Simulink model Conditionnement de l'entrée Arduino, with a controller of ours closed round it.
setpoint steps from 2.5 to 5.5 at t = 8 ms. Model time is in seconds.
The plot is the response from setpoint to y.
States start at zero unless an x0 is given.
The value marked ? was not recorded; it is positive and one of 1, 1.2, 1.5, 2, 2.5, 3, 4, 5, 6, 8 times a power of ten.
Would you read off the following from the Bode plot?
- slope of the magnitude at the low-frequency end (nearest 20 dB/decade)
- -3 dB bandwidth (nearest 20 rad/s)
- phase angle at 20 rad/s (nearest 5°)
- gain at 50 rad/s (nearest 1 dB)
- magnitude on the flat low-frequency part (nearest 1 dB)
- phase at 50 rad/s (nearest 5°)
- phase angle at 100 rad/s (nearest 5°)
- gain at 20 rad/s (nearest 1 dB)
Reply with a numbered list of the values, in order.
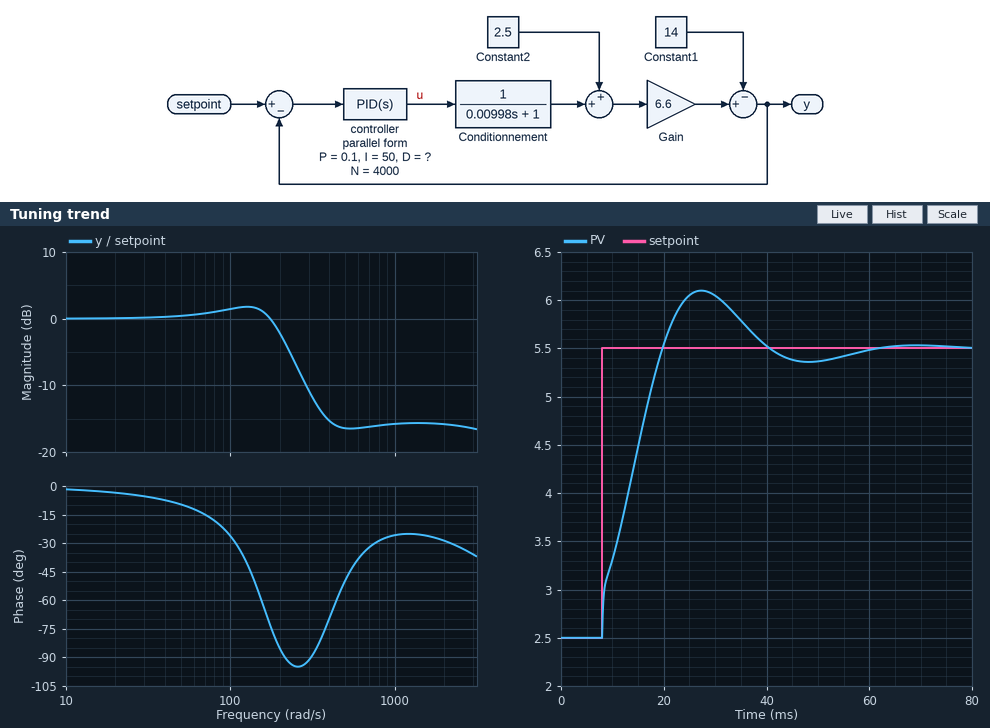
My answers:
1. 0 dB/decade
2. 200 rad/s
3. -5°
4. 0 dB
5. 0 dB
6. -10°
7. -25°
8. 0 dB
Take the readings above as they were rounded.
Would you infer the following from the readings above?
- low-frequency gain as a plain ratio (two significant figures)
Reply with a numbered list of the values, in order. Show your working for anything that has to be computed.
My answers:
1. 10^(0 / 20) = 1.0
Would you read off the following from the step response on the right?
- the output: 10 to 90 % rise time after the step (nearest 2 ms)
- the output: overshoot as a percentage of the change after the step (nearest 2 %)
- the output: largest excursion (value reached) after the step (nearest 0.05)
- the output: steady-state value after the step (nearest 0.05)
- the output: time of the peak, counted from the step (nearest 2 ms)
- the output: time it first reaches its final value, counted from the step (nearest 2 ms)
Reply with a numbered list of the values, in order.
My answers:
1. 10 ms
2. 20 %
3. 6.10
4. 5.50
5. 20 ms
6. 12 ms
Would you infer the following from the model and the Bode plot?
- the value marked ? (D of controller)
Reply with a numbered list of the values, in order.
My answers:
1. 0.0003
